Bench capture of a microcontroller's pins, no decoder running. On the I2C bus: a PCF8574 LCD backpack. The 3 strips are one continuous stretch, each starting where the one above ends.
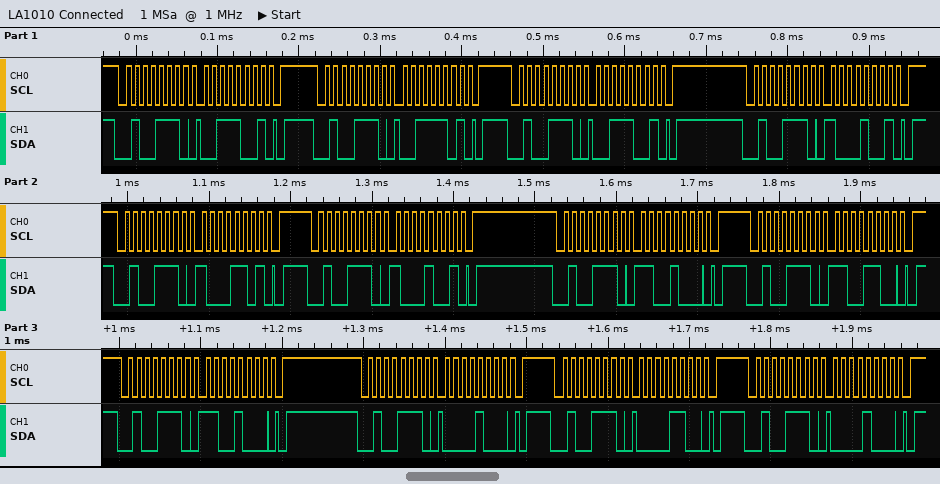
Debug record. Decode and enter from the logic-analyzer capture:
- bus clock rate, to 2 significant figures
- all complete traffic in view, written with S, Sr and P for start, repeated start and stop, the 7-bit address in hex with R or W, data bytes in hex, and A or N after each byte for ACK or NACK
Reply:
100 kHz
S 27W A 39 A P S 27W A 3D A P S 27W A 39 A P S 27W A 89 A P S 27W A 8D A P S 27W A 89 A P S 27W A C8 A P S 27W A CC A P S 27W A C8 A P S 27W A 08 A P S 27W A 0C A P S 27W A 08 A P
